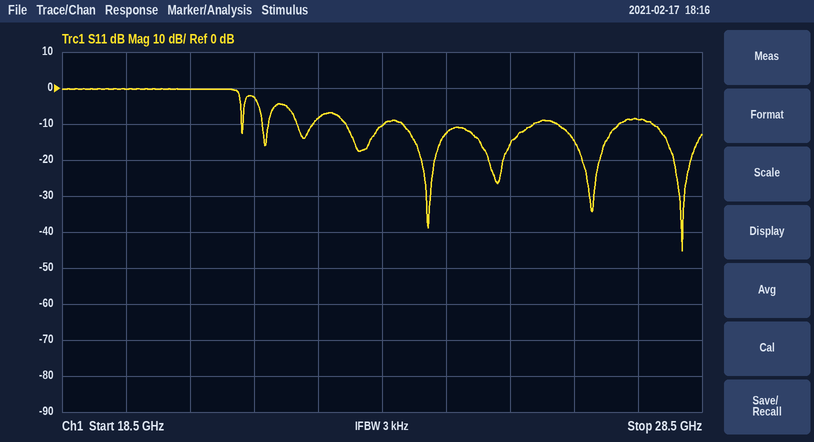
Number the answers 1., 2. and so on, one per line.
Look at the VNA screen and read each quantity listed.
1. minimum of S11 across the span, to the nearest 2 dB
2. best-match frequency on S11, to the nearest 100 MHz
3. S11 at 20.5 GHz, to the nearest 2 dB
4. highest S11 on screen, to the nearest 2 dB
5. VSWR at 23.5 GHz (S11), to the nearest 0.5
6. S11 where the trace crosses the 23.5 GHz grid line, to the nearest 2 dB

1. -46 dB
2. 28.2 GHz
3. 0 dB
4. 0 dB
5. 2.0
6. -10 dB
